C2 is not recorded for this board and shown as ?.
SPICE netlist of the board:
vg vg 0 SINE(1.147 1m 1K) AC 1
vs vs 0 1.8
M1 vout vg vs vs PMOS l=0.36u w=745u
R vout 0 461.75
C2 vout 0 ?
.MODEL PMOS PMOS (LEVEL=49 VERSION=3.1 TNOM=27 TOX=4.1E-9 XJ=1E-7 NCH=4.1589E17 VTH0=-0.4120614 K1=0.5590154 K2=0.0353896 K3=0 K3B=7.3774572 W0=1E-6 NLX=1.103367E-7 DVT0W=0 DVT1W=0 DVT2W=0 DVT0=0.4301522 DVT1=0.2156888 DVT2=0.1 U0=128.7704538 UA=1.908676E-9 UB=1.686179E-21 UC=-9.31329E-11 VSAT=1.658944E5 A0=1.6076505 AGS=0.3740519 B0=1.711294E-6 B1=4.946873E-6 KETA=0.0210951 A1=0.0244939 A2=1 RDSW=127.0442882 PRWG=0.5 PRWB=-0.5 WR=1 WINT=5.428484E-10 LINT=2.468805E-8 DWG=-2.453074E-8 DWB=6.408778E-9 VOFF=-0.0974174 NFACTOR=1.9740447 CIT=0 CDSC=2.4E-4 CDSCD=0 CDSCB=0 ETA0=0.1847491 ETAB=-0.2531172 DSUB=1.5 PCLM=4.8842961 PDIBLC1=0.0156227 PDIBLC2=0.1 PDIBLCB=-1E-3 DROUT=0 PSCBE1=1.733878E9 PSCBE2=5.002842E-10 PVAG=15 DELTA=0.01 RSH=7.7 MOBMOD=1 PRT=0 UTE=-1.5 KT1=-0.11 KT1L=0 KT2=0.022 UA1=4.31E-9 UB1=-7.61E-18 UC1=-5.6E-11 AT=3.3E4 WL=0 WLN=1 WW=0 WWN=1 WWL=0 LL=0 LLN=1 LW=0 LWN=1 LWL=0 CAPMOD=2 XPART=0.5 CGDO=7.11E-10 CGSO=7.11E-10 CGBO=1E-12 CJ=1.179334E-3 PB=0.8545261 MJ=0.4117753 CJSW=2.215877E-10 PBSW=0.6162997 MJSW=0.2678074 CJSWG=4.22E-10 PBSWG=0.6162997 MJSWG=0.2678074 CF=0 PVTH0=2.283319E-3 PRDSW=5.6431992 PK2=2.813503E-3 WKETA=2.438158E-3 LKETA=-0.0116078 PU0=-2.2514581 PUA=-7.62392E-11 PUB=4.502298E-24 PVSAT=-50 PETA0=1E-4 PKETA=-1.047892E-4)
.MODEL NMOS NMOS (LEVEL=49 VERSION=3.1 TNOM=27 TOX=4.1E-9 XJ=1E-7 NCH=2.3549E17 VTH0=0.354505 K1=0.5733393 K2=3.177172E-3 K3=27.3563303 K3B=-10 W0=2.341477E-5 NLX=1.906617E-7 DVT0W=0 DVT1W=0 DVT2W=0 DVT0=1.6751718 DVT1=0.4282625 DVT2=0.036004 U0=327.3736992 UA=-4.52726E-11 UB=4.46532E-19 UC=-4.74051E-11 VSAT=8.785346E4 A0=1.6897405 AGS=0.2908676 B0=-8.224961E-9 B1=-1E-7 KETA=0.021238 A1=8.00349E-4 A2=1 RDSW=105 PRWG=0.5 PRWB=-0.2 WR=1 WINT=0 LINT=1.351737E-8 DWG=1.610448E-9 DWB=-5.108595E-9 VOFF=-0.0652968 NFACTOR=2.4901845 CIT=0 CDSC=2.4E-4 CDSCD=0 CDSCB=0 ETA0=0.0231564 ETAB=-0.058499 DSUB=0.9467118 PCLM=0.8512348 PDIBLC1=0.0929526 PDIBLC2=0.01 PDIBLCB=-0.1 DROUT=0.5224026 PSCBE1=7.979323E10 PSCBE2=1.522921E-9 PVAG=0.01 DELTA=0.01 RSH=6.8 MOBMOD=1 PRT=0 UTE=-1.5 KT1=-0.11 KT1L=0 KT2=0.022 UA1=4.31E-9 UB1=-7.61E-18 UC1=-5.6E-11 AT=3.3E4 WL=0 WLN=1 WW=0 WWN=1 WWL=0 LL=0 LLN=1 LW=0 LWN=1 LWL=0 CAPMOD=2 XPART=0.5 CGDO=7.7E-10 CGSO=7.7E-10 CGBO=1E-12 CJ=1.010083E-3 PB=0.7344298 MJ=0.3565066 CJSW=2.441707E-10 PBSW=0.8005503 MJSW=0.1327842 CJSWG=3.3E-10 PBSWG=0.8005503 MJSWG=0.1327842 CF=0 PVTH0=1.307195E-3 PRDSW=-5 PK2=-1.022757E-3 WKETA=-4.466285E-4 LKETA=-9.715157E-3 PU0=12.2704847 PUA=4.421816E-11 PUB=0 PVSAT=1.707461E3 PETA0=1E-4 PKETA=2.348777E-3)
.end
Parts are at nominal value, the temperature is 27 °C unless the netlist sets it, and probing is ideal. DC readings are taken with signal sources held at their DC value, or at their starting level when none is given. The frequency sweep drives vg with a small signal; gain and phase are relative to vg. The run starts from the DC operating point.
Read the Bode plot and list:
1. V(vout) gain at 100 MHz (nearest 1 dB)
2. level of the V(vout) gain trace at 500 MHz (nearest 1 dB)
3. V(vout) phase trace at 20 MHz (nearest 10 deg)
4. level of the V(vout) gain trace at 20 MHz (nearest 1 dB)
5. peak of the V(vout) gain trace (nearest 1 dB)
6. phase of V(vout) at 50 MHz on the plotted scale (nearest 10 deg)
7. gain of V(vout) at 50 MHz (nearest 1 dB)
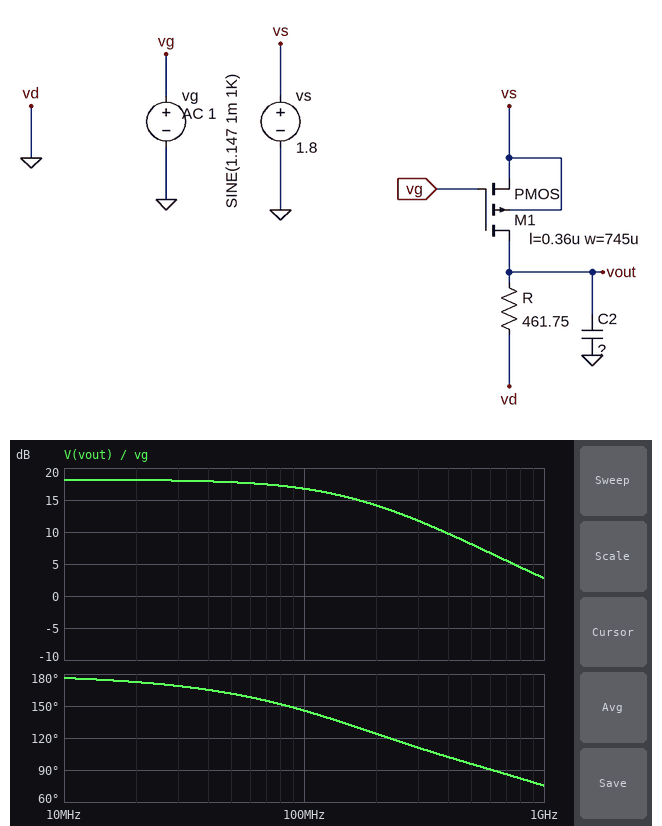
17 dB
8 dB
170 deg
18 dB
18 dB
160 deg
18 dB
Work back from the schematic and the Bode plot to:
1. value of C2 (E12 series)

1.5 pF
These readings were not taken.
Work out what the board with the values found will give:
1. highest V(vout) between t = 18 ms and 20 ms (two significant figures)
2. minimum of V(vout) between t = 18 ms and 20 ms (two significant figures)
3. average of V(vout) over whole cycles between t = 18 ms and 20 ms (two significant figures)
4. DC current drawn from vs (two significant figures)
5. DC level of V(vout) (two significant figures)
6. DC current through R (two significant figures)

960 mV
940 mV
950 mV
2.1 mA
950 mV
2.1 mA
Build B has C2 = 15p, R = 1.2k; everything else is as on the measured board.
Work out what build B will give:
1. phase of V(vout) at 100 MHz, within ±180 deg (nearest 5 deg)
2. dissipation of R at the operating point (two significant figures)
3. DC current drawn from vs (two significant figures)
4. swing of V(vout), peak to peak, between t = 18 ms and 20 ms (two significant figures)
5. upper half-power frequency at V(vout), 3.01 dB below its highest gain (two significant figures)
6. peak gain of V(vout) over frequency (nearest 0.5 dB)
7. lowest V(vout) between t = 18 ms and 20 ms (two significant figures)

130 deg
2.4 mW
1.4 mA
1.7 mV
100 MHz
-1.5 dB
1.7 V
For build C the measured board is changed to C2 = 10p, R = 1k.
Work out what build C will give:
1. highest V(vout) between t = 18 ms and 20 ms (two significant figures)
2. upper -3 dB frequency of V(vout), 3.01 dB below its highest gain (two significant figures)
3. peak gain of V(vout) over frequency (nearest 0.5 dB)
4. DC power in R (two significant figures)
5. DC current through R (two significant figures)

1.7 V
110 MHz
4.0 dB
2.8 mW
1.7 mA
